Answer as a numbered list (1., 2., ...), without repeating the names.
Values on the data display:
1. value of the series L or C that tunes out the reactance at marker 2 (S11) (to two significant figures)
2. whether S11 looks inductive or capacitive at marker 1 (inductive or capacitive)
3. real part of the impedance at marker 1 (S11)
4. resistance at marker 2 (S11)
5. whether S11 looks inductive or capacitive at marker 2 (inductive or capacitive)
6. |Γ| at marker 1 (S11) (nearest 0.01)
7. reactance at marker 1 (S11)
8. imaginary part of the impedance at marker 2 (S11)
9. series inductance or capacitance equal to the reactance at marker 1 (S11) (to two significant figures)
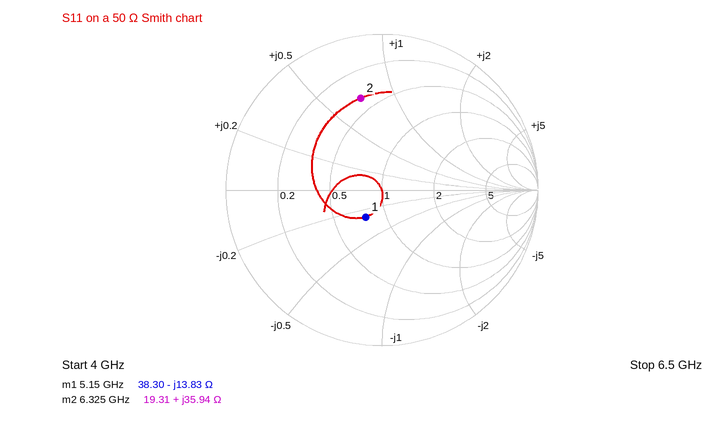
1. 700 fF
2. capacitive
3. 38.30 Ω
4. 19.31 Ω
5. inductive
6. 0.20
7. -13.83 Ω
8. +35.94 Ω
9. 2.2 pF
